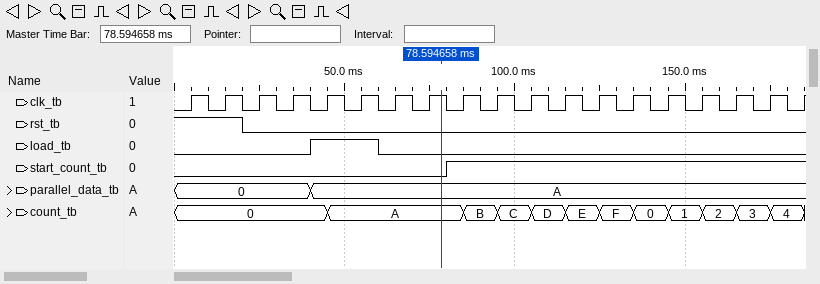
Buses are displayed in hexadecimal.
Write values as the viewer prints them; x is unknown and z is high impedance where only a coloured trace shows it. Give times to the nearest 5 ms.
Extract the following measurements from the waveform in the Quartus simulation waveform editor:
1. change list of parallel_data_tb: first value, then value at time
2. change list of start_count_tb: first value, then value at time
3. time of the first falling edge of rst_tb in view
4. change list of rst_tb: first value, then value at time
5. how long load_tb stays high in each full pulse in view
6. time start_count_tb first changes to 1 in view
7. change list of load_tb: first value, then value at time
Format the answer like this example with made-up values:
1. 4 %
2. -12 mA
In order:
1. 0, A at 40 ms
2. 0, 1 at 80 ms
3. 20 ms
4. 1, 0 at 20 ms
5. 20 ms
6. 80 ms
7. 0, 1 at 40 ms, 0 at 60 ms
